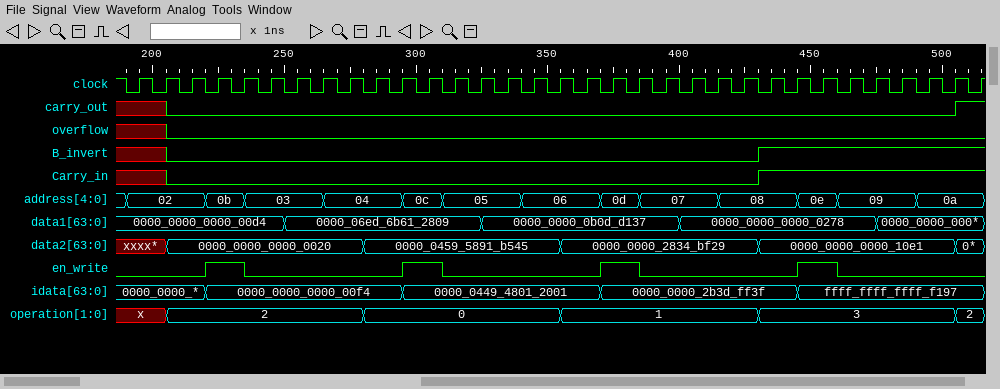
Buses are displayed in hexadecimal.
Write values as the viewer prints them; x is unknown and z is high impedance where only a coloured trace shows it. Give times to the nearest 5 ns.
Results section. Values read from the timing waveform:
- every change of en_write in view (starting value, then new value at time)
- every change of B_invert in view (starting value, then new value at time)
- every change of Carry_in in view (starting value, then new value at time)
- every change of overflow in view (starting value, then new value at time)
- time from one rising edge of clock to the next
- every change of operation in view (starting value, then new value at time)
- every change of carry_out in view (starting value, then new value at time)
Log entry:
0, 1 at 220 ns, 0 at 235 ns, 1 at 295 ns, 0 at 310 ns, 1 at 370 ns, 0 at 385 ns, 1 at 445 ns, 0 at 460 ns
x, 0 at 205 ns, 1 at 430 ns
x, 0 at 205 ns, 1 at 430 ns
x, 0 at 205 ns
10 ns
x, 2 at 205 ns, 0 at 280 ns, 1 at 355 ns, 3 at 430 ns, 2 at 505 ns
x, 0 at 205 ns, 1 at 505 ns
